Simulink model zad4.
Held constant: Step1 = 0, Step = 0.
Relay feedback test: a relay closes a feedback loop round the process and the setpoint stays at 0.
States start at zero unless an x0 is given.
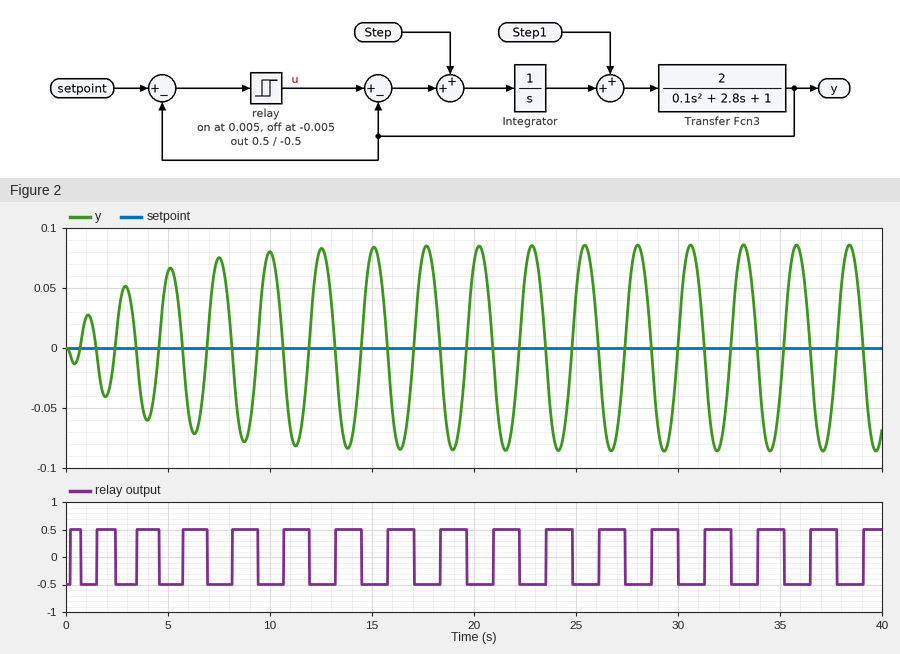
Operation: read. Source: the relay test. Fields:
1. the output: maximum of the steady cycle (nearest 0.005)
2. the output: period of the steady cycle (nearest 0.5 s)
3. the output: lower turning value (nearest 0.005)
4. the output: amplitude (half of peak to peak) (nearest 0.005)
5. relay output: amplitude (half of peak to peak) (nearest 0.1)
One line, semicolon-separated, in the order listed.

0.085; 2.5 s; -0.085; 0.085; 0.5
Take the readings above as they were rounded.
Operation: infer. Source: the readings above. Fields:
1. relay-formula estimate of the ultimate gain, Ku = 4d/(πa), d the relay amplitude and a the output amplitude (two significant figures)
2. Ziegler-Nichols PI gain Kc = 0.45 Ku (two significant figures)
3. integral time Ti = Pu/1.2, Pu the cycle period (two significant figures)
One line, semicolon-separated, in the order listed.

7.5; 3.4; 2.1 s
